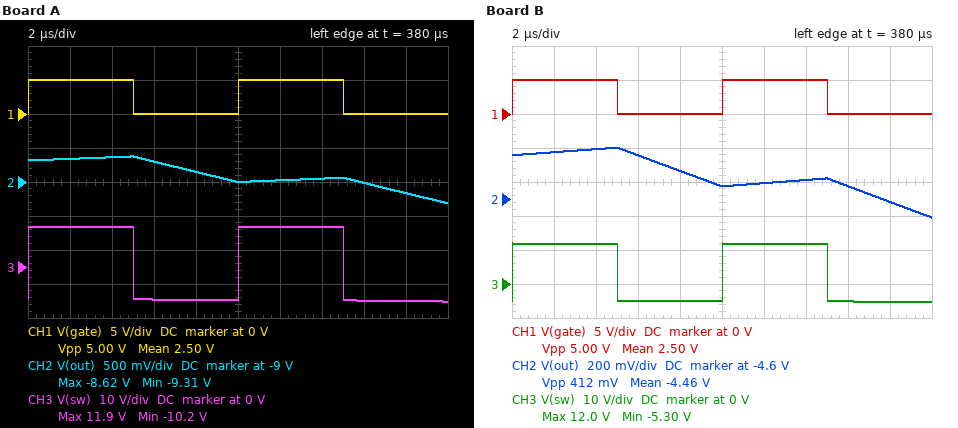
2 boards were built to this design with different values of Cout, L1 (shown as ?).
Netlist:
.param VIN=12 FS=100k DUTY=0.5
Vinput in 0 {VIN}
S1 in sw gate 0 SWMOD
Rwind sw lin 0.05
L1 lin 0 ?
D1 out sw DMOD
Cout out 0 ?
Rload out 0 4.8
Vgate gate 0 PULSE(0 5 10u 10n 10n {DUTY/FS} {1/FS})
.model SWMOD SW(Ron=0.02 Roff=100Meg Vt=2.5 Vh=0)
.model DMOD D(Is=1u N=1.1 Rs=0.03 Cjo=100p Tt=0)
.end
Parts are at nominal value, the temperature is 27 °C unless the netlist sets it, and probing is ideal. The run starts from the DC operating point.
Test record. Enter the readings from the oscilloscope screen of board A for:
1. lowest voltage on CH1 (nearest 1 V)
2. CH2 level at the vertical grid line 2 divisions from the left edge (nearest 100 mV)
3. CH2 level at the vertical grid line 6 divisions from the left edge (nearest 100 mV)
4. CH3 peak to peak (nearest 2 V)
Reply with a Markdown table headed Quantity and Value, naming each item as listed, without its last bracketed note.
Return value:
| Quantity | Value |
|---|---|
| lowest voltage on CH1 | 0 V |
| CH2 level at the vertical grid line 2 divisions from the left edge | -8.6 V |
| CH2 level at the vertical grid line 6 divisions from the left edge | -9.0 V |
| CH3 peak to peak | 22 V |
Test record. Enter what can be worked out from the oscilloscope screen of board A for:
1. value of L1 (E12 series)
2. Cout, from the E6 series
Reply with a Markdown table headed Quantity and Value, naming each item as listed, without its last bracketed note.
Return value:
| Quantity | Value |
|---|---|
| value of L1 | 100 µH |
| Cout, from the E6 series | 150 µF |
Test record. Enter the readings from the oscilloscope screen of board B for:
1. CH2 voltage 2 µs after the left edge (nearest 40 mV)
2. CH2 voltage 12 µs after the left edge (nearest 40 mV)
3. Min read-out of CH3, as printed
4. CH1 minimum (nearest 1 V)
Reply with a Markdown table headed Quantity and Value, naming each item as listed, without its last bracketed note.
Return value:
| Quantity | Value |
|---|---|
| CH2 voltage 2 µs after the left edge | -4.32 V |
| CH2 voltage 12 µs after the left edge | -4.52 V |
| Min read-out of CH3, as printed | -5.30 V |
| CH1 minimum | 0 V |
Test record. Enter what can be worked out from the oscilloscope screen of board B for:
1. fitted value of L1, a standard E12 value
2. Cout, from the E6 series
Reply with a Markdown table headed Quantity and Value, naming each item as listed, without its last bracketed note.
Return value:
| Quantity | Value |
|---|---|
| fitted value of L1, a standard E12 value | 330 µH |
| Cout, from the E6 series | 100 µF |
